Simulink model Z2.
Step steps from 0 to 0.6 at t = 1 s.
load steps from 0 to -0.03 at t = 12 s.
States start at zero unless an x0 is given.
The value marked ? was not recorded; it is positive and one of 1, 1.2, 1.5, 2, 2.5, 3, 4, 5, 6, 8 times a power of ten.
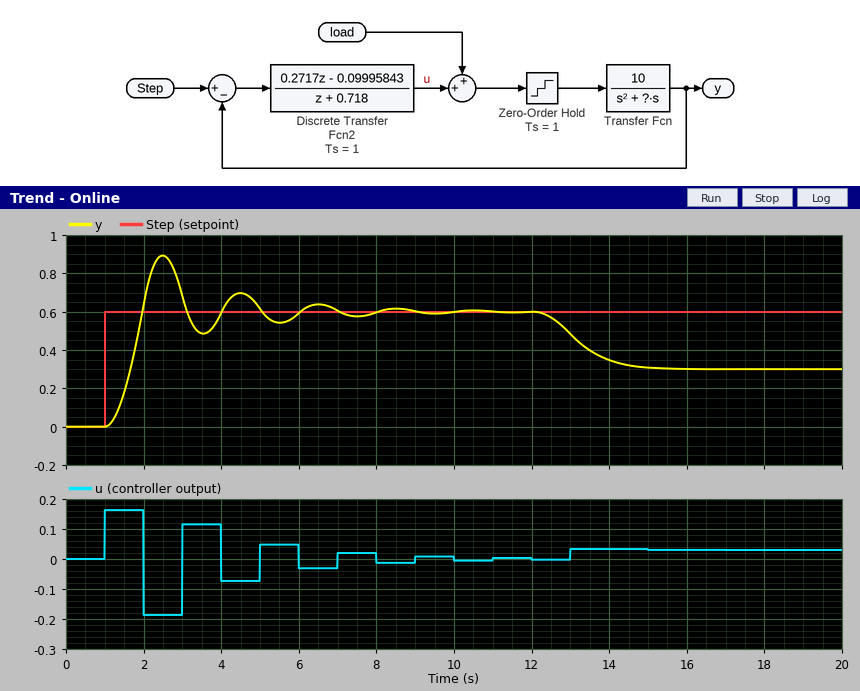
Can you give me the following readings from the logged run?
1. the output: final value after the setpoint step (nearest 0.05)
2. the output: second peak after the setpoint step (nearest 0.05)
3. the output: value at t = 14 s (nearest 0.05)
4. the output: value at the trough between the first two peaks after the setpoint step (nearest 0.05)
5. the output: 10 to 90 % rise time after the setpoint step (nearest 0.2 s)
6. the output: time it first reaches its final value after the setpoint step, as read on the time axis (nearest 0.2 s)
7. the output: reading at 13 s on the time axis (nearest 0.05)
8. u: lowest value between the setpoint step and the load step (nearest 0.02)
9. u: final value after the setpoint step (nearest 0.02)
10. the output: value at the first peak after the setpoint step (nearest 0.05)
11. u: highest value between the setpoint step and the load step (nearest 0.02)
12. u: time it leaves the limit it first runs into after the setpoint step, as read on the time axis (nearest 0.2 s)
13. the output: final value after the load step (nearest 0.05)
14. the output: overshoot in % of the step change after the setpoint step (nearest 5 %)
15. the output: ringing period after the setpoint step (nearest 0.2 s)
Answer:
0.60
0.70
0.35
0.50
0.6 s
2.0 s
0.50
-0.18
0.00
0.90
0.16
2.0 s
0.30
50 %
2.0 s
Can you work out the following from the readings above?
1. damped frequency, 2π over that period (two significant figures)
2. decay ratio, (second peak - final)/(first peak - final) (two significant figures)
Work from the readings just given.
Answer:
3.1 rad/s
0.33
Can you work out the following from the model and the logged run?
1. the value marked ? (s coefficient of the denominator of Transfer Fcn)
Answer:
0.8
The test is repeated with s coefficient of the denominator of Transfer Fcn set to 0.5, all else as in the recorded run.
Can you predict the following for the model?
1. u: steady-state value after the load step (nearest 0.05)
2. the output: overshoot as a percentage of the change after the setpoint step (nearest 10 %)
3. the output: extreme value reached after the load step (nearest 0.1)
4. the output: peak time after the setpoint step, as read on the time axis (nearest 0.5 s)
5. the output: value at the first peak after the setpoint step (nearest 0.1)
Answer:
0.05
70 %
0.3
2.5 s
1.0
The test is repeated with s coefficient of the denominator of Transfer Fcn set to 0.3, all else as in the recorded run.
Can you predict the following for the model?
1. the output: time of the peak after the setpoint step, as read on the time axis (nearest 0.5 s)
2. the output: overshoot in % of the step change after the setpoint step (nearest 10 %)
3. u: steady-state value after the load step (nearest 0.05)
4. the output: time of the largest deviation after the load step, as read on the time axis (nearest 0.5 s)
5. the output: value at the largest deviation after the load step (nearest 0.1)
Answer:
2.5 s
90 %
0.05
14.5 s
0.2
